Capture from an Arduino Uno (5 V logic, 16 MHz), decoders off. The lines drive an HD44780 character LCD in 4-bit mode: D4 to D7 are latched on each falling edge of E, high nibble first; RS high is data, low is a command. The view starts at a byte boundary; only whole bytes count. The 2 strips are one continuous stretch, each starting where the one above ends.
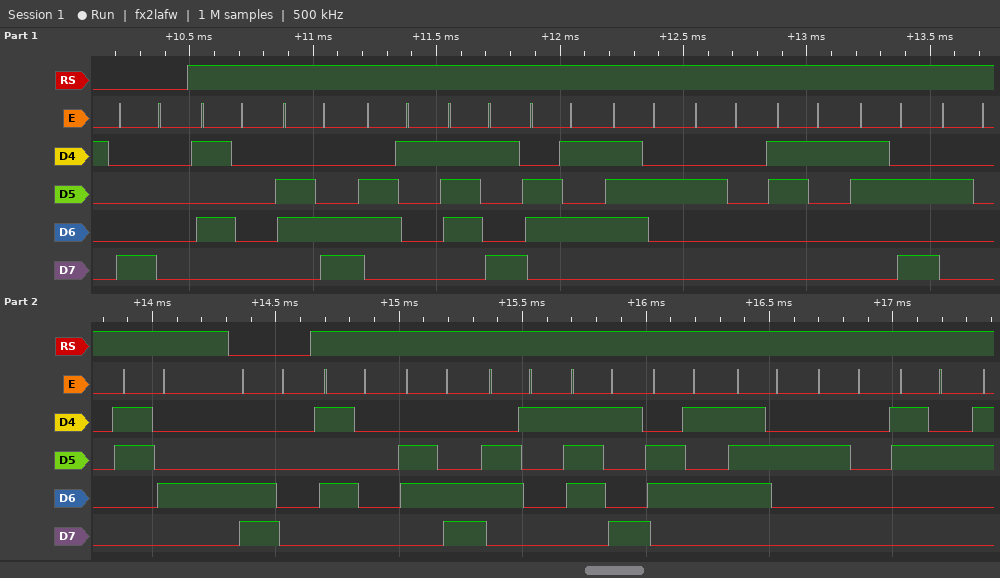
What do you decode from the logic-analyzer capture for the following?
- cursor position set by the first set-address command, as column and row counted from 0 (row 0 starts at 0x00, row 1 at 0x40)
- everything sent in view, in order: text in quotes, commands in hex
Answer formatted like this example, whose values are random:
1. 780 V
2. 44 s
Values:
1. column 0, row 0
2. 0x80 "Player 1: 4" 0xC0 "Player 2"
